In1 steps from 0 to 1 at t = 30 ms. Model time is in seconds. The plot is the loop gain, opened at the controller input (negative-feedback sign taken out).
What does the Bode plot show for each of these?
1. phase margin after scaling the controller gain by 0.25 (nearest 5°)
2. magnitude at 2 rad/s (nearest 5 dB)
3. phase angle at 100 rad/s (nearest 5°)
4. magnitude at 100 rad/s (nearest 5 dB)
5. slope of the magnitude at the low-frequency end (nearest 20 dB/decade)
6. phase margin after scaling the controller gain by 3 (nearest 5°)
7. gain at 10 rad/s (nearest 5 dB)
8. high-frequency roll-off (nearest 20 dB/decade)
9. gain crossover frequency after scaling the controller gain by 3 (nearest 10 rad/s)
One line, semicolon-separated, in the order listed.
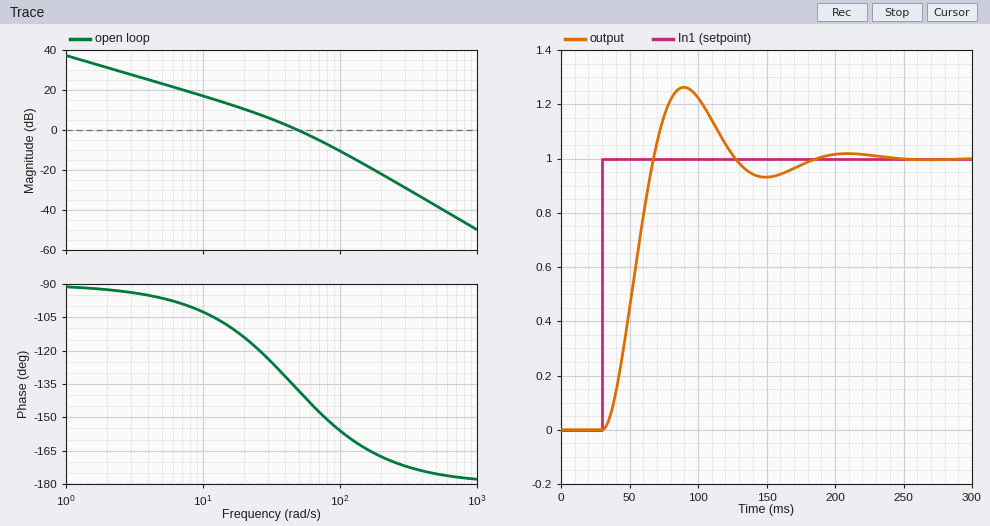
70°; 30 dB; -155°; -10 dB; -20 dB/decade; 25°; 15 dB; -40 dB/decade; 90 rad/s
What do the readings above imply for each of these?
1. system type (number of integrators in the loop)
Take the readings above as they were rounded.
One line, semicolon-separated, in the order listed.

1
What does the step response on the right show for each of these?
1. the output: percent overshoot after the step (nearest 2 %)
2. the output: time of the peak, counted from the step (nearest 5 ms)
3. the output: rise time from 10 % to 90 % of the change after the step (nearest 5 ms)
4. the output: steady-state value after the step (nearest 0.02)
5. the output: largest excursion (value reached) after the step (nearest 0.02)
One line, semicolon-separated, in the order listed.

26 %; 60 ms; 25 ms; 1.00; 1.26
